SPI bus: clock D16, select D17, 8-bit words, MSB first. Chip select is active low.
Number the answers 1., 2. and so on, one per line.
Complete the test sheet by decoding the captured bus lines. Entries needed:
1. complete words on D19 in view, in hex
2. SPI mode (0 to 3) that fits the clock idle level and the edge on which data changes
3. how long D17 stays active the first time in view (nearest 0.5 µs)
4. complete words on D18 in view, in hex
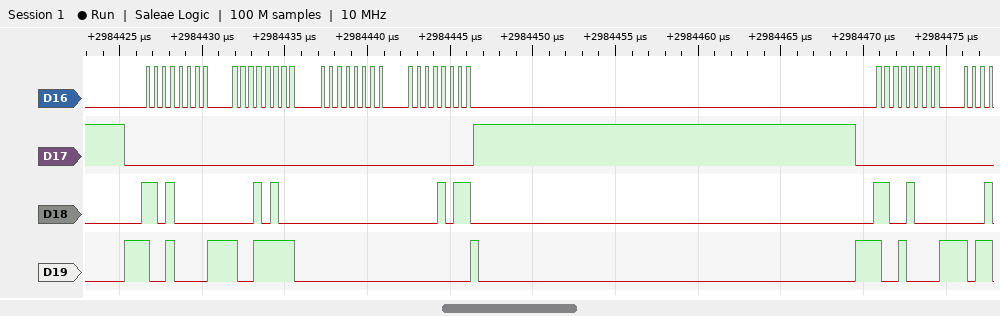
1. 90, 9F, 00, 00, 90
2. 0
3. 21 µs
4. D0, 14, 00, 0B, C8
